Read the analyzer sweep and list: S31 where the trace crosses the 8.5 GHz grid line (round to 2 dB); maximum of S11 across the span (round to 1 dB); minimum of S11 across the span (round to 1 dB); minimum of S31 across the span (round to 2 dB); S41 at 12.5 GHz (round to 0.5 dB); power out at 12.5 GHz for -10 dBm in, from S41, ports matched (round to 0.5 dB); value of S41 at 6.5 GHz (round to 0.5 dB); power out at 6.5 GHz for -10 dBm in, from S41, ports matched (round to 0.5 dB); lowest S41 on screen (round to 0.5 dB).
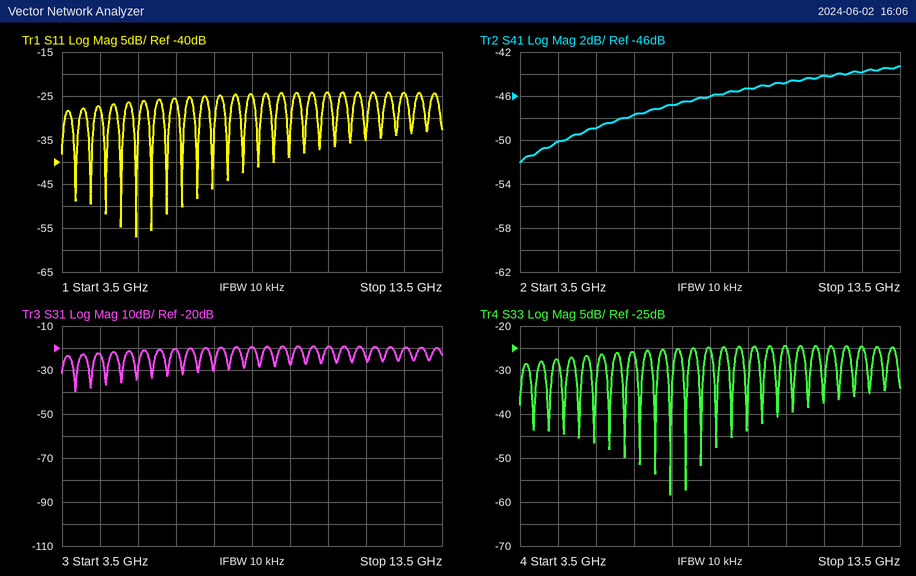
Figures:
-20 dB
-24 dB
-57 dB
-40 dB
-44.0 dB
-54.0 dBm
-47.5 dB
-57.5 dBm
-52.0 dB
